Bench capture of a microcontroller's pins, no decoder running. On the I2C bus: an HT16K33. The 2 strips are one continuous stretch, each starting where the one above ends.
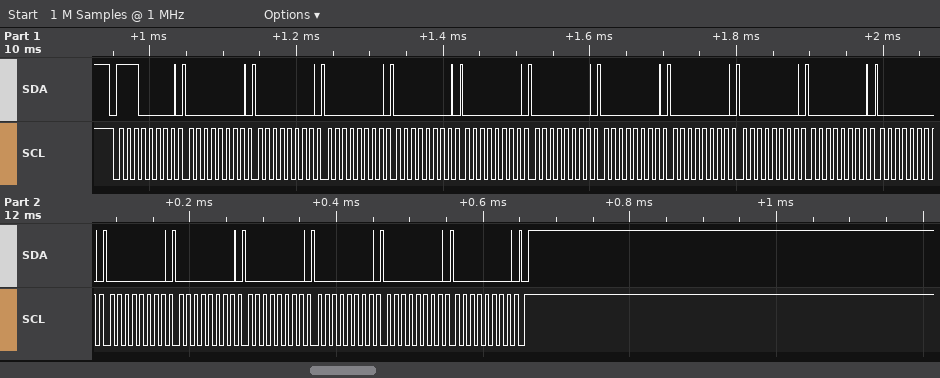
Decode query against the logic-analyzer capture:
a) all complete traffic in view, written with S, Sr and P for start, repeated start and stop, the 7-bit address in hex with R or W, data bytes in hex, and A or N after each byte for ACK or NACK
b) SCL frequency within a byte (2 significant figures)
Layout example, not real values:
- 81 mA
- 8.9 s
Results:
- S 70W A 00 A 00 A 00 A 00 A 00 A 00 A 00 A 00 A 00 A 00 A 00 A 00 A 00 A 00 A 00 A 00 A 00 A P
- 100 kHz
